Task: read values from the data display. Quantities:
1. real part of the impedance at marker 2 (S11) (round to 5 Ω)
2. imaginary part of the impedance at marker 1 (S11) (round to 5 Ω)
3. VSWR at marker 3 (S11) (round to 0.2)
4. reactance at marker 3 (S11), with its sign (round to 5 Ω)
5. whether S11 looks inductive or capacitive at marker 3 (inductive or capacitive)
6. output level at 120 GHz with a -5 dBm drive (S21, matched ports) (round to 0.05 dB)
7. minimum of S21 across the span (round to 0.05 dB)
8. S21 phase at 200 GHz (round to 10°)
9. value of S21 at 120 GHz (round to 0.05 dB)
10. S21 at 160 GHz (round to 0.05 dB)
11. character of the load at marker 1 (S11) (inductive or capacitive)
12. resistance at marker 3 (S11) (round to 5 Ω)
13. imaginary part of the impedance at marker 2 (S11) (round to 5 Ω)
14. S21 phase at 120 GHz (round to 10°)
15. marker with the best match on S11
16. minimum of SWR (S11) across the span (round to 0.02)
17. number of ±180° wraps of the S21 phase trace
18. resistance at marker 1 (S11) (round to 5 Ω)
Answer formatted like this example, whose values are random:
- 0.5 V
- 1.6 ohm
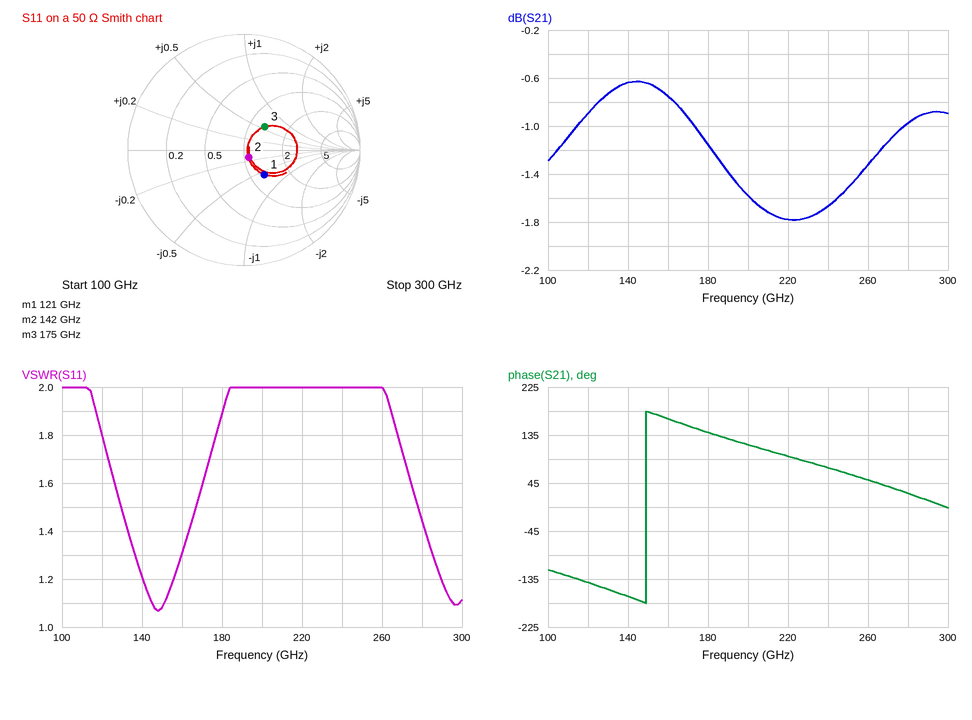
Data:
- 55 Ω
- -30 Ω
- 1.8
- +30 Ω
- inductive
- -5.90 dBm
- -1.80 dB
- 120°
- -0.90 dB
- -0.75 dB
- capacitive
- 65 Ω
- -5 Ω
- -140°
- marker 2
- 1.06
- 1
- 65 Ω
